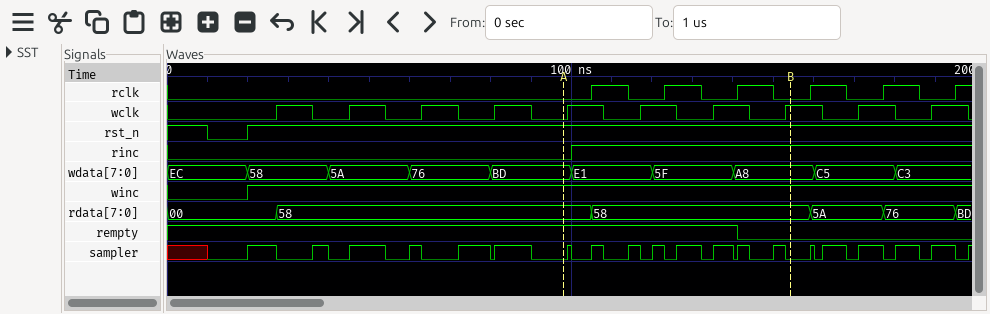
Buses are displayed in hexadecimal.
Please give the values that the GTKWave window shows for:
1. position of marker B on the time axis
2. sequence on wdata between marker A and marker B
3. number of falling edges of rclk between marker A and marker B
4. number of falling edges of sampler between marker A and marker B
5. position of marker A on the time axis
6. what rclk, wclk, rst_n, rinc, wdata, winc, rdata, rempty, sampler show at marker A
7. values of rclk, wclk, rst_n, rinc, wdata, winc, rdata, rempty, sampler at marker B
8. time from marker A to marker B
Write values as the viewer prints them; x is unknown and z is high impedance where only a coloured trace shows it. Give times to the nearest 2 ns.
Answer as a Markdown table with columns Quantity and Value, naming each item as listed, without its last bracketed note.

| Quantity | Value |
|---|---|
| position of marker B on the time axis | 154 ns |
| sequence on wdata between marker A and marker B | BD, E1, 5F, A8 |
| number of falling edges of rclk between marker A and marker B | 3 |
| number of falling edges of sampler between marker A and marker B | 8 |
| position of marker A on the time axis | 98 ns |
| what rclk, wclk, rst_n, rinc, wdata, winc, rdata, rempty, sampler show at marker A | rclk=0, wclk=0, rst_n=1, rinc=0, wdata=BD, winc=1, rdata=58, rempty=1, sampler=0 |
| values of rclk, wclk, rst_n, rinc, wdata, winc, rdata, rempty, sampler at marker B | rclk=0, wclk=1, rst_n=1, rinc=1, wdata=A8, winc=1, rdata=58, rempty=0, sampler=0 |
| time from marker A to marker B | 56 ns |
